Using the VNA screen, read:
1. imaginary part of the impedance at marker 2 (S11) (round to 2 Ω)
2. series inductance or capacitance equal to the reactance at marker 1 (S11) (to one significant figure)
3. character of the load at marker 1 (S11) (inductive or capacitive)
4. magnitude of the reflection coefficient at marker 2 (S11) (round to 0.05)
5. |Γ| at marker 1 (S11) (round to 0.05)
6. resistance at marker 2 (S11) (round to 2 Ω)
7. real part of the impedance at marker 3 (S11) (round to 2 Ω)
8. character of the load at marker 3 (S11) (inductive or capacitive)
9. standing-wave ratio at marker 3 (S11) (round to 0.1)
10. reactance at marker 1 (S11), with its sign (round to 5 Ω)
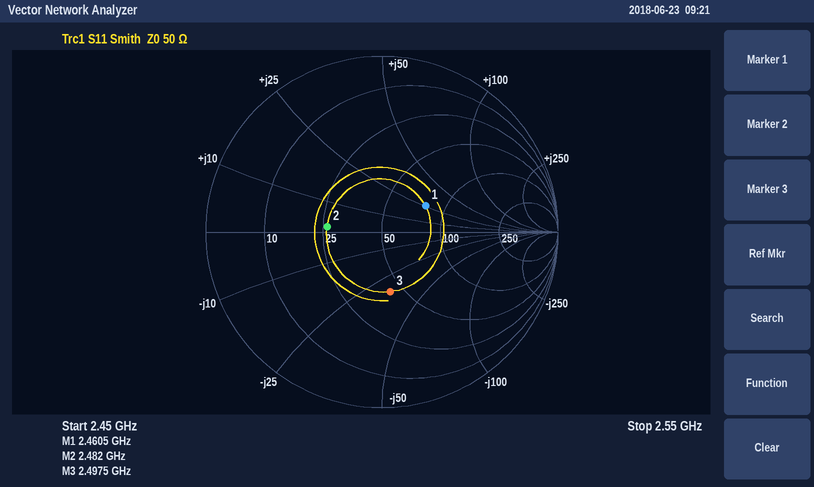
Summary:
+2 Ω
2 nH
inductive
0.30
0.30
26 Ω
44 Ω
capacitive
2.0
+25 Ω
